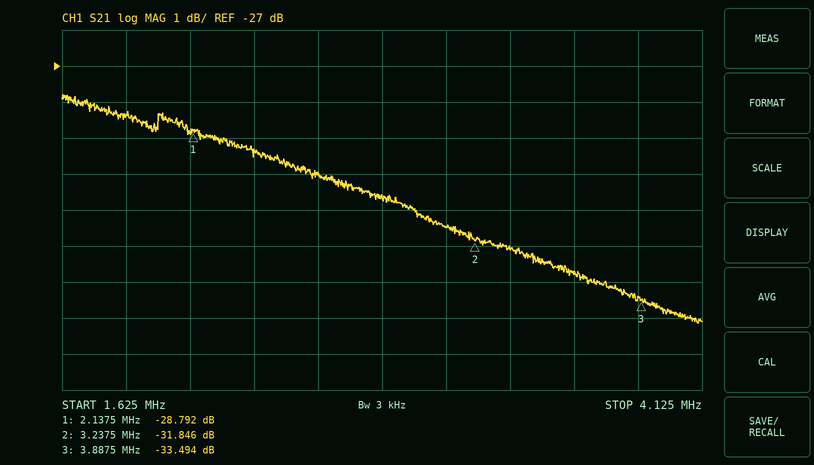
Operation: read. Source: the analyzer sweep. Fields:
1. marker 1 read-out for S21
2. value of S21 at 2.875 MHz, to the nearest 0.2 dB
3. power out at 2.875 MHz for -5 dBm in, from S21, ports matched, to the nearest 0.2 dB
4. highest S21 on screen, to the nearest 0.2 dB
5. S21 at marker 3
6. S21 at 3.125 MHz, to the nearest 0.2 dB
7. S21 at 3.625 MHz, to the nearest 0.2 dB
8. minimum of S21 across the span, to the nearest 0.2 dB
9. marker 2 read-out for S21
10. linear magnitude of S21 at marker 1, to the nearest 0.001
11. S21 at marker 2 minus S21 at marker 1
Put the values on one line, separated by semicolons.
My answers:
-28.792 dB; -30.6 dB; -35.6 dBm; -27.8 dB; -33.494 dB; -31.4 dB; -32.8 dB; -34.2 dB; -31.846 dB; 0.036; -3.054 dB
